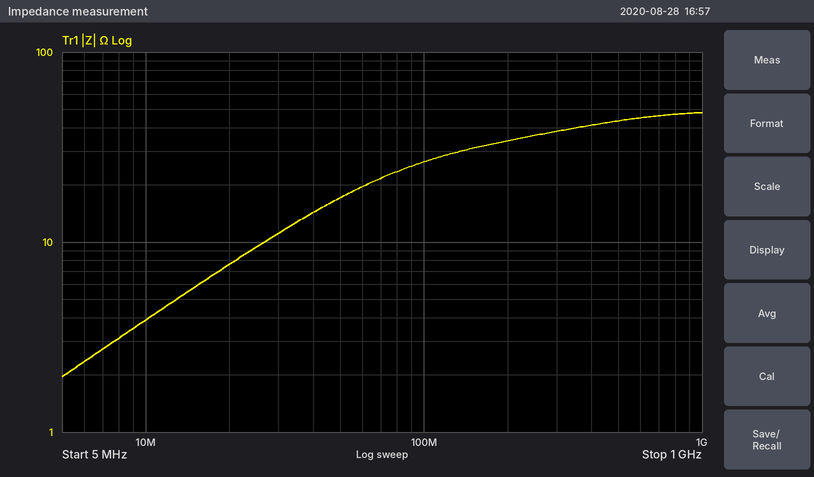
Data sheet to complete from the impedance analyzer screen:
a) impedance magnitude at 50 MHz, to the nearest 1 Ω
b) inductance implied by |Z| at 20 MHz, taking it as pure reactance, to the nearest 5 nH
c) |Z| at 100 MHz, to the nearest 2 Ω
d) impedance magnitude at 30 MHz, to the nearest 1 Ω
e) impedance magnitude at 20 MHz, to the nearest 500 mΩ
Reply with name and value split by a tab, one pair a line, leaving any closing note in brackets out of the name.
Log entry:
impedance magnitude at 50 MHz, to the nearest 1 Ω	17 Ω
inductance implied by |Z| at 20 MHz, taking it as pure reactance, to the nearest 5 nH	60 nH
|Z| at 100 MHz, to the nearest 2 Ω	26 Ω
impedance magnitude at 30 MHz, to the nearest 1 Ω	11 Ω
impedance magnitude at 20 MHz, to the nearest 500 mΩ	7.5 Ω
